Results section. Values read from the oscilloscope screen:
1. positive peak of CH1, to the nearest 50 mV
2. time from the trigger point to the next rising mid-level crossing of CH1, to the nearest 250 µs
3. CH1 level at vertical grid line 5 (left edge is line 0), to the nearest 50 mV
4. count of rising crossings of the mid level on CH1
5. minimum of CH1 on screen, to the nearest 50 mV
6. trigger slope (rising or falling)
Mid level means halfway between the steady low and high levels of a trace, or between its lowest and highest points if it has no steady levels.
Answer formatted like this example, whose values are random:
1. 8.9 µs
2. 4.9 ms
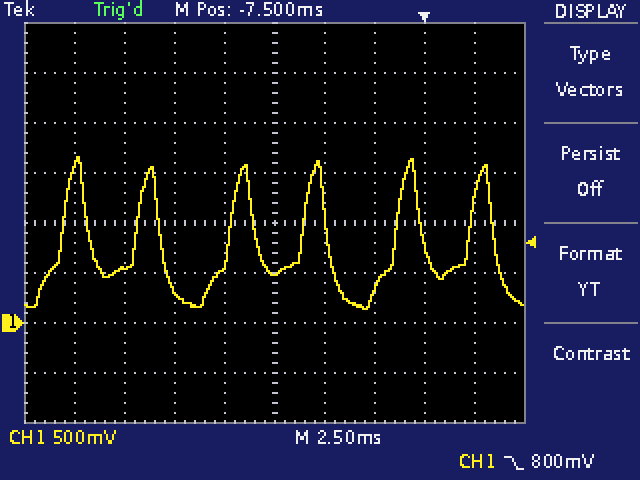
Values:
1. 1.65 V
2. 2.25 ms
3. 500 mV
4. 6
5. 150 mV
6. falling
